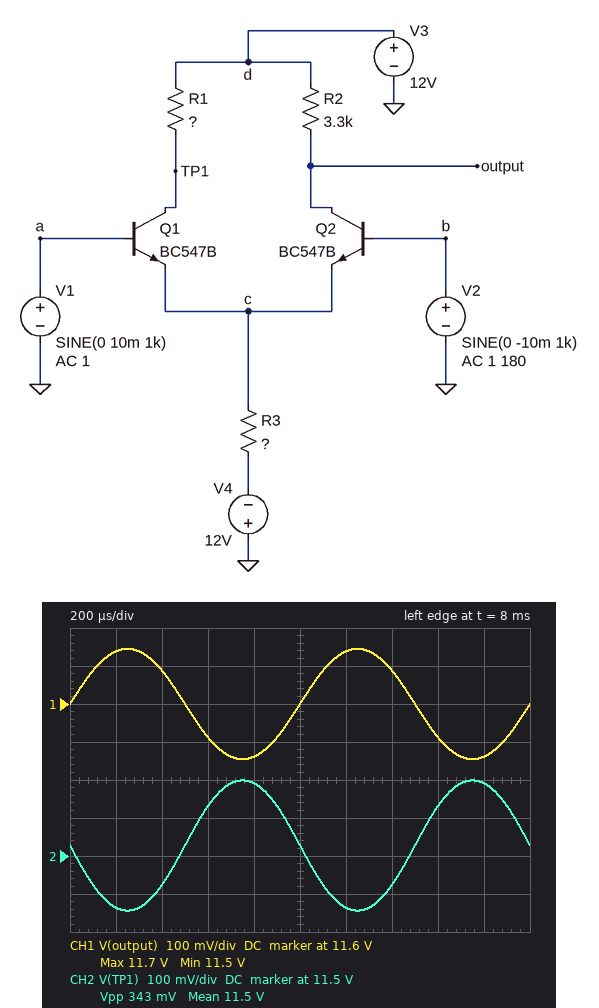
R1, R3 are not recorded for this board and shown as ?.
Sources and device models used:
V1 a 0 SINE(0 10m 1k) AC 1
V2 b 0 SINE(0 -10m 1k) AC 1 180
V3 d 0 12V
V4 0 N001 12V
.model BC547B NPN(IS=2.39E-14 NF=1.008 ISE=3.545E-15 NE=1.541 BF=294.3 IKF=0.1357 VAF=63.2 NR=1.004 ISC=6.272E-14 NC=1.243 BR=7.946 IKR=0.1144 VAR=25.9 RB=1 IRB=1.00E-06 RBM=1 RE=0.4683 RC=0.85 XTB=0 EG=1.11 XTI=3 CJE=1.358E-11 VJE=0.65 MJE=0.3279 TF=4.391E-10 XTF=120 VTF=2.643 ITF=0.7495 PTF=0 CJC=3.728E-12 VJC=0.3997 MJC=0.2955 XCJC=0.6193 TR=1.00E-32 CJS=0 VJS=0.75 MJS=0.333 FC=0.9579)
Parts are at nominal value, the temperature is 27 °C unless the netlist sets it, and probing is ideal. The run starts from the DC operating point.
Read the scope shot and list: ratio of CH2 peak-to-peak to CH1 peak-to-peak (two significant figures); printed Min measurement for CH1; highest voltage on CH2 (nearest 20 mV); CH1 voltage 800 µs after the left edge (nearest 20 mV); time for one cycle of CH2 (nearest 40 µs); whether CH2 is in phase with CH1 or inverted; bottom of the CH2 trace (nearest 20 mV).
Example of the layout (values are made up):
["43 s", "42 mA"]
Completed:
["1.2", "11.5 V", "11.70 V", "11.46 V", "1.00 ms", "inverted", "11.36 V"]
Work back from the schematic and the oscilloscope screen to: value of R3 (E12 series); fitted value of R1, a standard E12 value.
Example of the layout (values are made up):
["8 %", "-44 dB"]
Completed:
["47 kΩ", "3.9 kΩ"]
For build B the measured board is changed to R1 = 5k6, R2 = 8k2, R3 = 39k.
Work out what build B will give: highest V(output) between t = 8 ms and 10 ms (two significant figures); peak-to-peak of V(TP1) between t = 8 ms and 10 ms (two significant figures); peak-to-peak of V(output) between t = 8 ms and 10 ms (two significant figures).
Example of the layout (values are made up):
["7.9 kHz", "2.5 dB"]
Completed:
["11 V", "590 mV", "860 mV"]
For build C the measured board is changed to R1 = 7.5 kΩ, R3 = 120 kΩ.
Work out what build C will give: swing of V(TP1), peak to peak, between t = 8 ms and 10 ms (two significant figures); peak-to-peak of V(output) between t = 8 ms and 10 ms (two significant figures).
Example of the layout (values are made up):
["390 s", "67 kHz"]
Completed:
["260 mV", "110 mV"]
